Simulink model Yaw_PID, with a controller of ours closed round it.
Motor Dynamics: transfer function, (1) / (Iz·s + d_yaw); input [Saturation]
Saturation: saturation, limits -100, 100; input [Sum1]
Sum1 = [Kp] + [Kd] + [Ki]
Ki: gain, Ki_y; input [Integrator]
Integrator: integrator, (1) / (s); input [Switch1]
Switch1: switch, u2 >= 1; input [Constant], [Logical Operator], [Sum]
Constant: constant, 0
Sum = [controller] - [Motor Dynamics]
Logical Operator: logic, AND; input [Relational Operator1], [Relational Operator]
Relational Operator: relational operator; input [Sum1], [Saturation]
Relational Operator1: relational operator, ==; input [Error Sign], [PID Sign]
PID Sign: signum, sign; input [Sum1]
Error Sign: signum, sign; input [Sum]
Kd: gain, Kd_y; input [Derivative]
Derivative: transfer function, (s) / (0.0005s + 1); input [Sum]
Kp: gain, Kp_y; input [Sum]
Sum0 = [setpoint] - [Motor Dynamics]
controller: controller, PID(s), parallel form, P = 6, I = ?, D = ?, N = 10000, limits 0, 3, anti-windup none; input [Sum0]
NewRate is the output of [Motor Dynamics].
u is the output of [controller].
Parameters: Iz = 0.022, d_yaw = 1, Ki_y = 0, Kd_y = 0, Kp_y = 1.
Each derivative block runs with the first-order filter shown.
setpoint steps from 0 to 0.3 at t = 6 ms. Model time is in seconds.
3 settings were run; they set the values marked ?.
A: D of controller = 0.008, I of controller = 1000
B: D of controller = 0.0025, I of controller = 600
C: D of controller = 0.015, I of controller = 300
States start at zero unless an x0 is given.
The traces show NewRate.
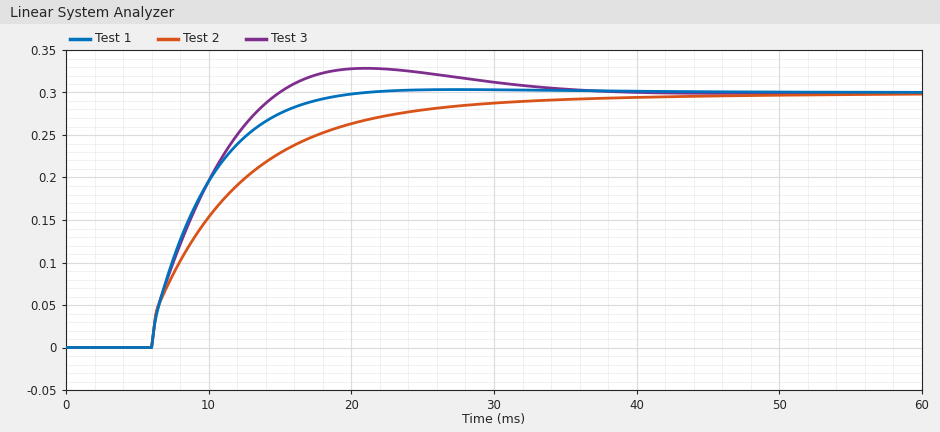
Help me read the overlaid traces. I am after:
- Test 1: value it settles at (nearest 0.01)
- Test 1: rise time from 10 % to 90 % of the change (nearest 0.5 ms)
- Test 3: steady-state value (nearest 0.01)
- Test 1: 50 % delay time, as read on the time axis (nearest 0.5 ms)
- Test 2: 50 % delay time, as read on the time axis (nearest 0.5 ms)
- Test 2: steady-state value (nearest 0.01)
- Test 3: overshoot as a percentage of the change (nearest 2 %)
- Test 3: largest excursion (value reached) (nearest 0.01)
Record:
0.30
8.0 ms
0.30
8.5 ms
10.0 ms
0.30
10 %
0.33
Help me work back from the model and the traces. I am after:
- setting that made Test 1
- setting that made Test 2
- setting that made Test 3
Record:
B
C
A
